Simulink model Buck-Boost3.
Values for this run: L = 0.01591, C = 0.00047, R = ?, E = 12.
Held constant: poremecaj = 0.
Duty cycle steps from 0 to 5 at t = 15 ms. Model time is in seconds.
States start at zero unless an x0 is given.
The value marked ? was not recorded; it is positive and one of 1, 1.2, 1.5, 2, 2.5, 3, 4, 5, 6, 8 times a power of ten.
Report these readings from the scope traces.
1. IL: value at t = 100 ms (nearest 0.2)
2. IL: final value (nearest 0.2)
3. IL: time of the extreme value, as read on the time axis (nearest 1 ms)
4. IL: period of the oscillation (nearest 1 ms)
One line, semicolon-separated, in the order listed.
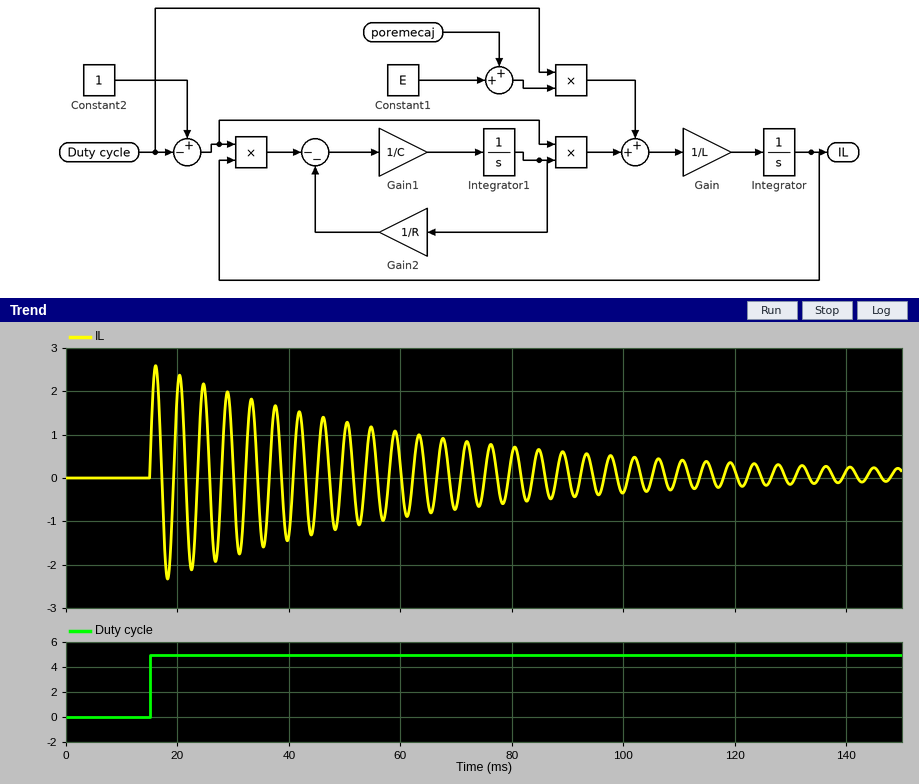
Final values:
-0.4; 0.0; 16 ms; 4 ms
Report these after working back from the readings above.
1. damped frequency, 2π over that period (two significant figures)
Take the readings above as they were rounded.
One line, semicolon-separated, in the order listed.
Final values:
1.6 rad/ms
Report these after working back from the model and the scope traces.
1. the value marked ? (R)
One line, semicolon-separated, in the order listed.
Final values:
50
